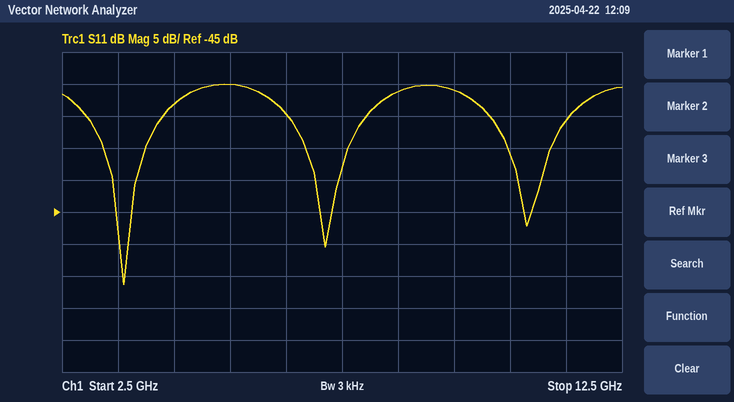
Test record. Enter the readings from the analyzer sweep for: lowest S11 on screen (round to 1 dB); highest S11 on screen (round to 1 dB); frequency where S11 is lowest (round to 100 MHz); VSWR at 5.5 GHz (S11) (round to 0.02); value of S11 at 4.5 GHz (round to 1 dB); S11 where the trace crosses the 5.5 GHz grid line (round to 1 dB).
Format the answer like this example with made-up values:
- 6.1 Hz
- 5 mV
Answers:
- -56 dB
- -25 dB
- 3.6 GHz
- 1.12
- -28 dB
- -25 dB
